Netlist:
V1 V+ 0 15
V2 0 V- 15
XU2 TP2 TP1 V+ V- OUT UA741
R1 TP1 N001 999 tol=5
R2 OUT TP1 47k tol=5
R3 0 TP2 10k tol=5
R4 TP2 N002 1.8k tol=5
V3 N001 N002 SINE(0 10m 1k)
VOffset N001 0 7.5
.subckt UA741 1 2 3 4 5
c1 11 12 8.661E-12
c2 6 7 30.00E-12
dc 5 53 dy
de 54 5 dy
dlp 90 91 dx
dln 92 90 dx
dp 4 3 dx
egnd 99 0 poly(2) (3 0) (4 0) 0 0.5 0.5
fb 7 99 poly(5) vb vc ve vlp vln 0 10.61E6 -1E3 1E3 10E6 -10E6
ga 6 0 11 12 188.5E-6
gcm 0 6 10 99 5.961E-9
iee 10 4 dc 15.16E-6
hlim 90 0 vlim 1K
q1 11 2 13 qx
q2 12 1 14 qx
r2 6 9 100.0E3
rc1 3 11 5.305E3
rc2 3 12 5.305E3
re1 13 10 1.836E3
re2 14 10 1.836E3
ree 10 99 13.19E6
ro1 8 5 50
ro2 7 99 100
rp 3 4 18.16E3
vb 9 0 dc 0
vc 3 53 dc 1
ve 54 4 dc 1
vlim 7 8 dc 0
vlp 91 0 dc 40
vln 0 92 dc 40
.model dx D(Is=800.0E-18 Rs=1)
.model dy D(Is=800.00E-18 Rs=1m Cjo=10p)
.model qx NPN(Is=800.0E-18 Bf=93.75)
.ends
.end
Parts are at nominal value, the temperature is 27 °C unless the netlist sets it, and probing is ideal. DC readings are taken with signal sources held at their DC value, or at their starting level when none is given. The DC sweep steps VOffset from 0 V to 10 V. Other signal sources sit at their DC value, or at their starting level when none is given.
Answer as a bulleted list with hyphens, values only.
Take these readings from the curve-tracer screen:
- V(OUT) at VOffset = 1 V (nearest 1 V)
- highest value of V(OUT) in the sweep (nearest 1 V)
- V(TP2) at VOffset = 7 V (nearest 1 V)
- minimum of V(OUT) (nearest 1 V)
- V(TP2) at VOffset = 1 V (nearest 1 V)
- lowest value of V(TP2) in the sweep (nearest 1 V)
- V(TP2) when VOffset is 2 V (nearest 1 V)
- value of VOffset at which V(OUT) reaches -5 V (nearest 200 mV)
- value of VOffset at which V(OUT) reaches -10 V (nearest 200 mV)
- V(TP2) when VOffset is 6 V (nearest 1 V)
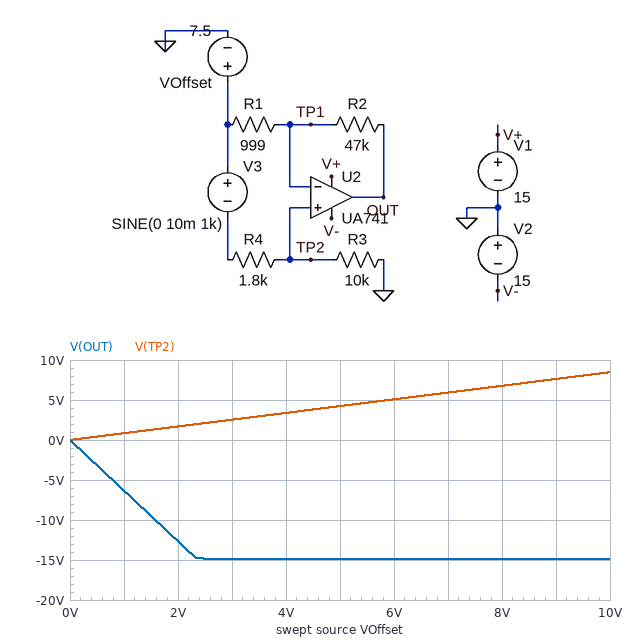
- -6 V
- 0 V
- 6 V
- -15 V
- 1 V
- 0 V
- 2 V
- 800 mV
- 1.6 V
- 5 V
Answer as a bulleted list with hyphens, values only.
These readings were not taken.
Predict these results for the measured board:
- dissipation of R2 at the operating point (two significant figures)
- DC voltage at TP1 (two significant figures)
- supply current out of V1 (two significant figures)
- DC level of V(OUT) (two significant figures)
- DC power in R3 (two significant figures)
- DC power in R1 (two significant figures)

- 10 mW
- 7.0 V
- 1.7 mA
- -15 V
- 4.0 mW
- 220 µW
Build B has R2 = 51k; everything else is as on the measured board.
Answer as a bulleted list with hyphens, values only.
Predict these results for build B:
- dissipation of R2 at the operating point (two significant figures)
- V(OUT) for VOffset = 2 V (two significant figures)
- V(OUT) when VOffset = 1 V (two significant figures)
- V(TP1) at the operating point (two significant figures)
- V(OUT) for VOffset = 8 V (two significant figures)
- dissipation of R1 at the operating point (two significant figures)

- 9.4 mW
- -14 V
- -6.9 V
- 7.1 V
- -15 V
- 180 µW
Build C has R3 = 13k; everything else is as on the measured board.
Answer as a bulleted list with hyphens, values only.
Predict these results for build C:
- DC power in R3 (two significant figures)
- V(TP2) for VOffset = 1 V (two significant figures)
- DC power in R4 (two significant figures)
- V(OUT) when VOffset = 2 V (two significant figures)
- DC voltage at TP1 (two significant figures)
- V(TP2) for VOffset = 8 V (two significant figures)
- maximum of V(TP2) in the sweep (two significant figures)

- 3.3 mW
- 880 mV
- 460 µW
- -9.7 V
- 7.0 V
- 7.0 V
- 8.8 V
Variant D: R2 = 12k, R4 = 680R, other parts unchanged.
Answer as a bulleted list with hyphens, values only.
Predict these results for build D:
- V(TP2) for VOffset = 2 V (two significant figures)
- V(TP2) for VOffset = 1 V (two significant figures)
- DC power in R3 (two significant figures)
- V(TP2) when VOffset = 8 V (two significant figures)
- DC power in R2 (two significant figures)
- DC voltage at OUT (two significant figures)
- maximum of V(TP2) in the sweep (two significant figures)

- 1.9 V
- 940 mV
- 4.9 mW
- 7.5 V
- 2.7 mW
- 1.3 V
- 9.4 V
